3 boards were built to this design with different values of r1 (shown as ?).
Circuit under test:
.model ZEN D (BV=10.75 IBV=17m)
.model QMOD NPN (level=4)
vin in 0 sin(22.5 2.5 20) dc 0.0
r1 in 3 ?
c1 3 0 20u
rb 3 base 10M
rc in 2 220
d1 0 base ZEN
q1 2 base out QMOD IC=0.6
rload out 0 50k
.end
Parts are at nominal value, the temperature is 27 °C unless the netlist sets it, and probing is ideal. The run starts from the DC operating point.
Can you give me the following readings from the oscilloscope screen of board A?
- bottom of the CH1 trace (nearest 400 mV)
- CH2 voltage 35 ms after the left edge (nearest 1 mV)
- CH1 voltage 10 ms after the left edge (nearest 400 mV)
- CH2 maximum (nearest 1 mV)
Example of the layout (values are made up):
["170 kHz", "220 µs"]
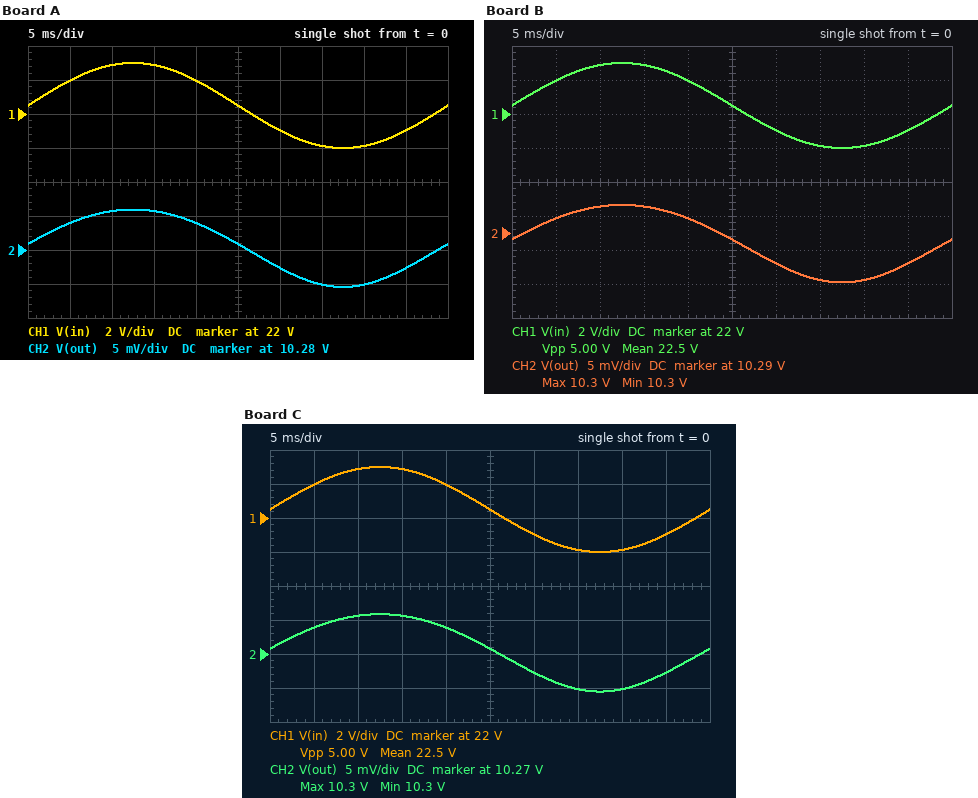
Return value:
["20.0 V", "10.275 V", "24.8 V", "10.286 V"]
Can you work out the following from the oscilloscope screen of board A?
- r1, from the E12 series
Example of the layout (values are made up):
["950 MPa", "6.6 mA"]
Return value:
["0.015 Ω"]
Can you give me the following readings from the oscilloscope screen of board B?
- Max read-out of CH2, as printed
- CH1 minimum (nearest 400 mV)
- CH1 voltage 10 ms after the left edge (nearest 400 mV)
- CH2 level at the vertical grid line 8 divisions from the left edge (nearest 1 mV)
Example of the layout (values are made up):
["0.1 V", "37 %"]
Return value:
["10.3 V", "20.0 V", "24.8 V", "10.283 V"]
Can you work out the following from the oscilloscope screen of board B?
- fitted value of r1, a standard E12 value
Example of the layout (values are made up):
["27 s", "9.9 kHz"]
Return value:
["8.2 mΩ"]
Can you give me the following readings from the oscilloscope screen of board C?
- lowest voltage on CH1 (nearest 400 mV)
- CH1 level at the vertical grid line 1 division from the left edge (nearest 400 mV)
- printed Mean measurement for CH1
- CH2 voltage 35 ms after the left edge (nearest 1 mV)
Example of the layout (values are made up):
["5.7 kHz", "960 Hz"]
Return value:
["20.0 V", "24.0 V", "22.5 V", "10.265 V"]
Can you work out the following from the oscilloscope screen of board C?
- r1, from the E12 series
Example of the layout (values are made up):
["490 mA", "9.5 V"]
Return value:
["0.027 Ω"]
